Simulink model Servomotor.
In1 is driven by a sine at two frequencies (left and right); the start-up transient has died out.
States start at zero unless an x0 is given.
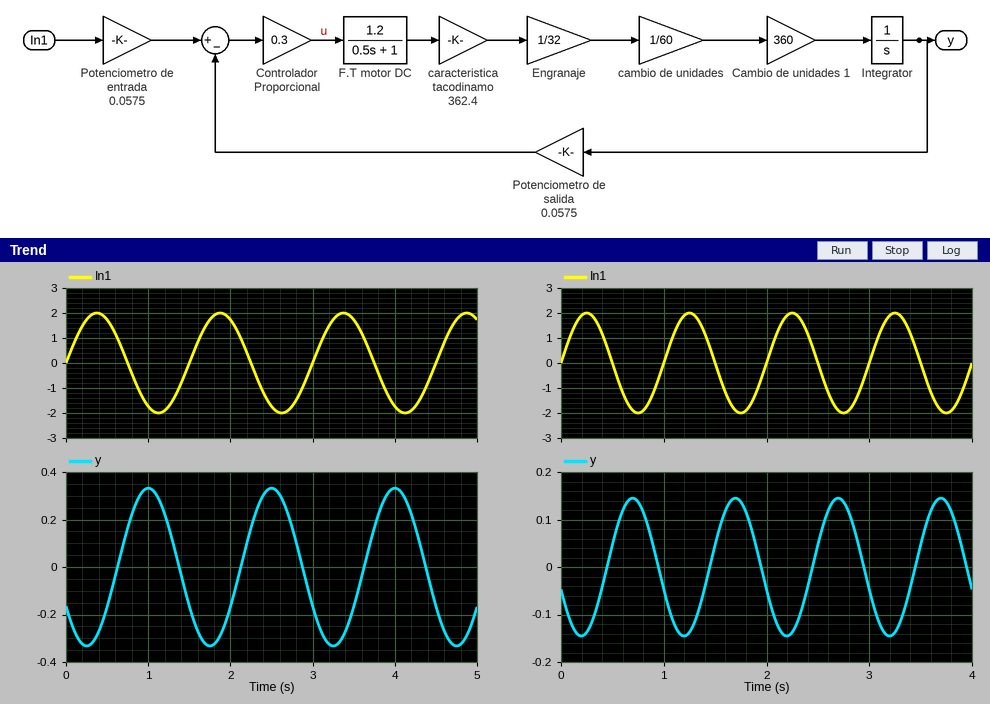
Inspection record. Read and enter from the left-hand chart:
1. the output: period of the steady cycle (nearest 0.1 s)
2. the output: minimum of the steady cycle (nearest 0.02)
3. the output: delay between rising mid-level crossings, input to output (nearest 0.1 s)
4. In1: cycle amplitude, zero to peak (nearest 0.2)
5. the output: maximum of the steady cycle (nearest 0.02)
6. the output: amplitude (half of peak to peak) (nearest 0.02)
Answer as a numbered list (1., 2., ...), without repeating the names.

1. 1.5 s
2. -0.34
3. 0.6 s
4. 2.0
5. 0.34
6. 0.34
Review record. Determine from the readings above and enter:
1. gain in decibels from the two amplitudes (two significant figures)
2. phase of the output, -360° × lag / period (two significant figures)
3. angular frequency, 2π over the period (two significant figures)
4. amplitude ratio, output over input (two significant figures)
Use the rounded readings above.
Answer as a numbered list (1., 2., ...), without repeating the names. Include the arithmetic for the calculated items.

1. 20 log10(0.34 / 2) = -15 dB
2. -360 × 0.6 / 1.5 = -140°
3. 2π / 1.5 = 4.2 rad/s
4. 0.34 / 2 = 0.17
